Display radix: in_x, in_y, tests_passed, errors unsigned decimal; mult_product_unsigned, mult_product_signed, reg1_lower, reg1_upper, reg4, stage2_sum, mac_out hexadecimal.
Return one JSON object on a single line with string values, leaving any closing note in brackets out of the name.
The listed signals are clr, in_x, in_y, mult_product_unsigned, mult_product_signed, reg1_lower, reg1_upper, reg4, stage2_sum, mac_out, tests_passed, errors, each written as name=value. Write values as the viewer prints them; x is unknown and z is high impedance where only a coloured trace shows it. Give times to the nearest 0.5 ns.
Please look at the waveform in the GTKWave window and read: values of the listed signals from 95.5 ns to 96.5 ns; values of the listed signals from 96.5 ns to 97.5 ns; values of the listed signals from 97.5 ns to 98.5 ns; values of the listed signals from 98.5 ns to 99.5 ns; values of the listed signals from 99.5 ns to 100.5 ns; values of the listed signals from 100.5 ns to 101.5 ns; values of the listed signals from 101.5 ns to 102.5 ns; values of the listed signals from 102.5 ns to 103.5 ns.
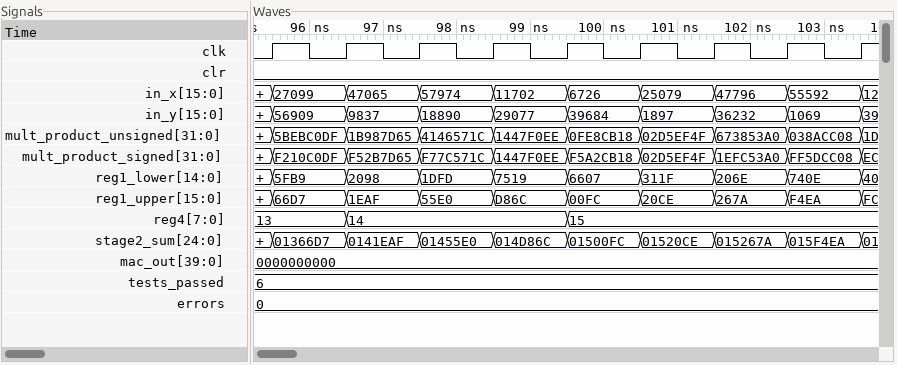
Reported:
{"values of the listed signals from 95.5 ns to 96.5 ns": "clr=0, in_x=27099, in_y=56909, mult_product_unsigned=5BEBC0DF, mult_product_signed=F210C0DF, reg1_lower=5FB9, reg1_upper=66D7, reg4=13, stage2_sum=01366D7, mac_out=0000000000, tests_passed=6, errors=0", "values of the listed signals from 96.5 ns to 97.5 ns": "clr=0, in_x=47065, in_y=9837, mult_product_unsigned=1B987D65, mult_product_signed=F52B7D65, reg1_lower=2098, reg1_upper=1EAF, reg4=14, stage2_sum=0141EAF, mac_out=0000000000, tests_passed=6, errors=0", "values of the listed signals from 97.5 ns to 98.5 ns": "clr=0, in_x=57974, in_y=18890, mult_product_unsigned=4146571C, mult_product_signed=F77C571C, reg1_lower=1DFD, reg1_upper=55E0, reg4=14, stage2_sum=01455E0, mac_out=0000000000, tests_passed=6, errors=0", "values of the listed signals from 98.5 ns to 99.5 ns": "clr=0, in_x=11702, in_y=29077, mult_product_unsigned=1447F0EE, mult_product_signed=1447F0EE, reg1_lower=7519, reg1_upper=D86C, reg4=14, stage2_sum=014D86C, mac_out=0000000000, tests_passed=6, errors=0", "values of the listed signals from 99.5 ns to 100.5 ns": "clr=0, in_x=6726, in_y=39684, mult_product_unsigned=0FE8CB18, mult_product_signed=F5A2CB18, reg1_lower=6607, reg1_upper=00FC, reg4=15, stage2_sum=01500FC, mac_out=0000000000, tests_passed=6, errors=0", "values of the listed signals from 100.5 ns to 101.5 ns": "clr=0, in_x=25079, in_y=1897, mult_product_unsigned=02D5EF4F, mult_product_signed=02D5EF4F, reg1_lower=311F, reg1_upper=20CE, reg4=15, stage2_sum=01520CE, mac_out=0000000000, tests_passed=6, errors=0", "values of the listed signals from 101.5 ns to 102.5 ns": "clr=0, in_x=47796, in_y=36232, mult_product_unsigned=673853A0, mult_product_signed=1EFC53A0, reg1_lower=206E, reg1_upper=267A, reg4=15, stage2_sum=015267A, mac_out=0000000000, tests_passed=6, errors=0", "values of the listed signals from 102.5 ns to 103.5 ns": "clr=0, in_x=55592, in_y=1069, mult_product_unsigned=038ACC08, mult_product_signed=FF5DCC08, reg1_lower=740E, reg1_upper=F4EA, reg4=15, stage2_sum=015F4EA, mac_out=0000000000, tests_passed=6, errors=0"}
